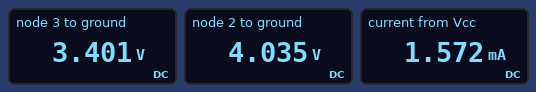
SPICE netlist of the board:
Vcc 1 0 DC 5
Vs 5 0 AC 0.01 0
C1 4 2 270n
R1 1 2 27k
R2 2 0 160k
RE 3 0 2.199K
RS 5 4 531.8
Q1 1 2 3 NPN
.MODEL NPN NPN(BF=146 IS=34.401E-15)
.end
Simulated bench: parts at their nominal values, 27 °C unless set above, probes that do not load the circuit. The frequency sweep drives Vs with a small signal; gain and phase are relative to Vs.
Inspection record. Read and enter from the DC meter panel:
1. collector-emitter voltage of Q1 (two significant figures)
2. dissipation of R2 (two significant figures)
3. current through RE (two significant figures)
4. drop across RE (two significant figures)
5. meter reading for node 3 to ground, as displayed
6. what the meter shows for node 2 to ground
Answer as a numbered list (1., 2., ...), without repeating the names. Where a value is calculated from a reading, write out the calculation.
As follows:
1. 5 V - 3.401 V = 1.6 V
2. (4.035 V)^2 / 160 kΩ = 100 µW
3. (3.401 V) / 2.199 kΩ = 1.5 mA
4. 3.401 V = 3.4 V
5. 3.401 V
6. 4.035 V
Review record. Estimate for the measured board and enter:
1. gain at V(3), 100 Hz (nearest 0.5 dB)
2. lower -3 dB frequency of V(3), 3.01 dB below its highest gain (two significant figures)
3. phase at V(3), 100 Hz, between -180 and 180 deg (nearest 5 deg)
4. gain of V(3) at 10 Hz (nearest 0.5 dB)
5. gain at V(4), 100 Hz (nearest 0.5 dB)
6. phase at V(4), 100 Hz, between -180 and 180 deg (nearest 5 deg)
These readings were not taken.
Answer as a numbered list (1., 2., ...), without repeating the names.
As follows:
1. -0.5 dB
2. 27 Hz
3. 15 deg
4. -9.5 dB
5. 0 dB
6. 0 deg
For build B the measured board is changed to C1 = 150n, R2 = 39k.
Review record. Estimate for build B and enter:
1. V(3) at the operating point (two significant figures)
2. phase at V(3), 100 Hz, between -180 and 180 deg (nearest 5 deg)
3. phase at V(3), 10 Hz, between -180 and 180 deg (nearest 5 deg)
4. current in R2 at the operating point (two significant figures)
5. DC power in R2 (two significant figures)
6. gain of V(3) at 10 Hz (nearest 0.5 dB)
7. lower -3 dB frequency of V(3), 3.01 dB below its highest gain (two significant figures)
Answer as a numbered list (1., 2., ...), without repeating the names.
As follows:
1. 2.2 V
2. 35 deg
3. 80 deg
4. 73 µA
5. 210 µW
6. -17.0 dB
7. 67 Hz
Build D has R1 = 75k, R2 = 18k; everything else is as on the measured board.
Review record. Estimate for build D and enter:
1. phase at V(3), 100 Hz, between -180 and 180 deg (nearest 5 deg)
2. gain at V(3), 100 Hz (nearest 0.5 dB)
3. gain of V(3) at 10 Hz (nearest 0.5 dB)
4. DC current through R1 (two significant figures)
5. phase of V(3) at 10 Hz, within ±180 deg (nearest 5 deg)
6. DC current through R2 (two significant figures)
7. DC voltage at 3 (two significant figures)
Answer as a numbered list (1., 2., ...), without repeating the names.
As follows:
1. 20 deg
2. -1.5 dB
3. -13.5 dB
4. 54 µA
5. 75 deg
6. 53 µA
7. 370 mV
